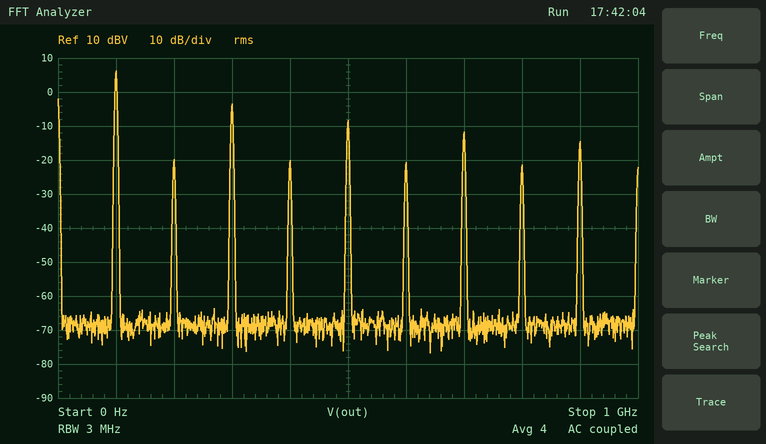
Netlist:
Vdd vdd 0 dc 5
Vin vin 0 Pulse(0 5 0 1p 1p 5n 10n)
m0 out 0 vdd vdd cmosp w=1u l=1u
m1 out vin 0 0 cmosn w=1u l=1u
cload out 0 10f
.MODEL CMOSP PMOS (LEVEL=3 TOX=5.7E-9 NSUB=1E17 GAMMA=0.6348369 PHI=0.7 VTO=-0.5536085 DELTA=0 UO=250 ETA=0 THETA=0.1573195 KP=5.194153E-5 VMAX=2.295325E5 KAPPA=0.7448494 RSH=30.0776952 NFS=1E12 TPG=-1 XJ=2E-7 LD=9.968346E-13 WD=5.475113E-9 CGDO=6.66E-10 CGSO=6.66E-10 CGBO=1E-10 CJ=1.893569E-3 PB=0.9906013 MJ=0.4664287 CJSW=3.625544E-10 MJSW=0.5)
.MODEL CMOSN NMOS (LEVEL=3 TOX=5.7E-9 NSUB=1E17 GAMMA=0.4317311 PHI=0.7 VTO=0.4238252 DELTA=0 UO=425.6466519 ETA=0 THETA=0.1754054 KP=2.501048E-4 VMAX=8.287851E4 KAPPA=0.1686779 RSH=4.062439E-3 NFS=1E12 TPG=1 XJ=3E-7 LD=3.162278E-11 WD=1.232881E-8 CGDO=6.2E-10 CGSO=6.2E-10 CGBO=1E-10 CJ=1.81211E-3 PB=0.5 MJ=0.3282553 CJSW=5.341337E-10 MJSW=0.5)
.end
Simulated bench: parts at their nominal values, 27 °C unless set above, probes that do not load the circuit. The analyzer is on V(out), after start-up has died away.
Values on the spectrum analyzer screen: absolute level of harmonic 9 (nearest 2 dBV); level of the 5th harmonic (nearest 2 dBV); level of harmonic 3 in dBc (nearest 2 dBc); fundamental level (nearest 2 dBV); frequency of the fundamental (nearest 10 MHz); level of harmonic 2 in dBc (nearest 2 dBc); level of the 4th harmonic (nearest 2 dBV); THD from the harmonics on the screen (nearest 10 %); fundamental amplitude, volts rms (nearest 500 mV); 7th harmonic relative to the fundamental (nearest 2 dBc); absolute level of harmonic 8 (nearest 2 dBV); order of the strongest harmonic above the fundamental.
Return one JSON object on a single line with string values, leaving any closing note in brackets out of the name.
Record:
{"absolute level of harmonic 9": "-14 dBV", "level of the 5th harmonic": "-8 dBV", "level of harmonic 3 in dBc": "-10 dBc", "fundamental level": "6 dBV", "frequency of the fundamental": "100 MHz", "level of harmonic 2 in dBc": "-26 dBc", "level of the 4th harmonic": "-20 dBV", "THD from the harmonics on the screen": "40 %", "fundamental amplitude, volts rms": "2.0 V", "7th harmonic relative to the fundamental": "-18 dBc", "absolute level of harmonic 8": "-22 dBV", "order of the strongest harmonic above the fundamental": "3"}
